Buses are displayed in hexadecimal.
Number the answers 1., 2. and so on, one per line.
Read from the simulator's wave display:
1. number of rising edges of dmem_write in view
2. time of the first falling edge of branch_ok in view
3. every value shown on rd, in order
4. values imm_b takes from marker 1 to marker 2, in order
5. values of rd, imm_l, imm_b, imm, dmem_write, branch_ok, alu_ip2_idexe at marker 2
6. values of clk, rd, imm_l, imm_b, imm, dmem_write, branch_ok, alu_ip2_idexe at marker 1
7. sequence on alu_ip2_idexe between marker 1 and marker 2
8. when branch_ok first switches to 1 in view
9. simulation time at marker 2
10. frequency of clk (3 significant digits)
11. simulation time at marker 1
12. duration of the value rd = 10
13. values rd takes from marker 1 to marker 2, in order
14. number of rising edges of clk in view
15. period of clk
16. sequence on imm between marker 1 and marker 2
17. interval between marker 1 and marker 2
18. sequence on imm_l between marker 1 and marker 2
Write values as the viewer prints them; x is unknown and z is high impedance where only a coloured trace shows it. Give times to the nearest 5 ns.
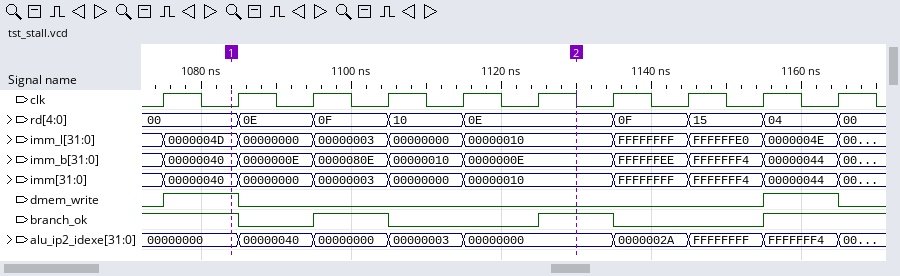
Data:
1. 2
2. 1085 ns
3. 00, 0E, 0F, 10, 0E, 0F, 15, 04, 00
4. 00000040, 0000000E, 0000080E, 00000010, 0000000E
5. rd=0E, imm_l=00000010, imm_b=0000000E, imm=00000010, dmem_write=0, branch_ok=1, alu_ip2_idexe=00000000
6. clk=0, rd=00, imm_l=0000004D, imm_b=00000040, imm=00000040, dmem_write=1, branch_ok=1, alu_ip2_idexe=00000000
7. 00000000, 00000040, 00000000, 00000003, 00000000
8. 1095 ns
9. 1130 ns
10. 100 MHz
11. 1085 ns
12. 10 ns
13. 00, 0E, 0F, 10, 0E
14. 10
15. 10 ns
16. 00000040, 00000000, 00000003, 00000000, 00000010
17. 45 ns
18. 0000004D, 00000000, 00000003, 00000000, 00000010
